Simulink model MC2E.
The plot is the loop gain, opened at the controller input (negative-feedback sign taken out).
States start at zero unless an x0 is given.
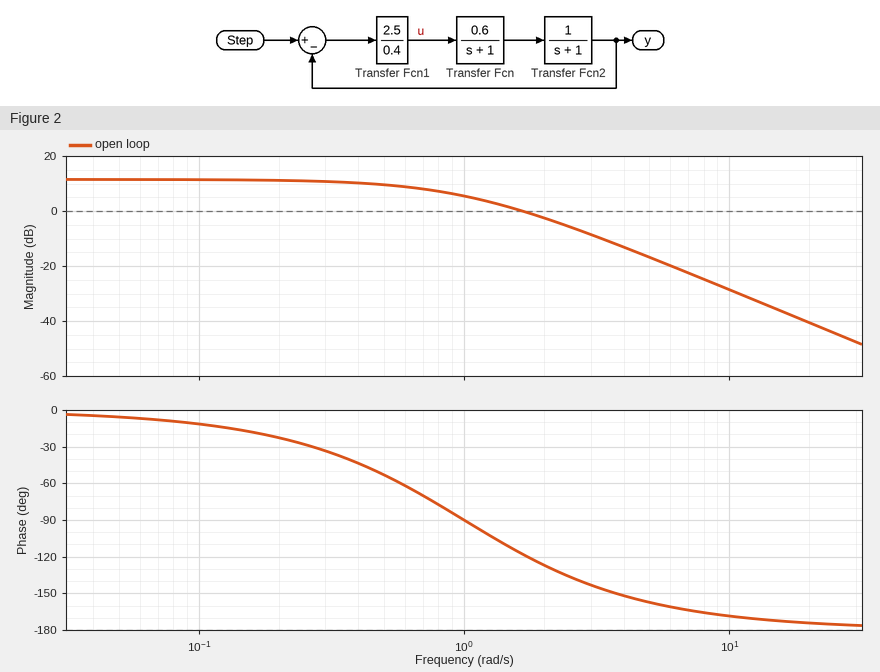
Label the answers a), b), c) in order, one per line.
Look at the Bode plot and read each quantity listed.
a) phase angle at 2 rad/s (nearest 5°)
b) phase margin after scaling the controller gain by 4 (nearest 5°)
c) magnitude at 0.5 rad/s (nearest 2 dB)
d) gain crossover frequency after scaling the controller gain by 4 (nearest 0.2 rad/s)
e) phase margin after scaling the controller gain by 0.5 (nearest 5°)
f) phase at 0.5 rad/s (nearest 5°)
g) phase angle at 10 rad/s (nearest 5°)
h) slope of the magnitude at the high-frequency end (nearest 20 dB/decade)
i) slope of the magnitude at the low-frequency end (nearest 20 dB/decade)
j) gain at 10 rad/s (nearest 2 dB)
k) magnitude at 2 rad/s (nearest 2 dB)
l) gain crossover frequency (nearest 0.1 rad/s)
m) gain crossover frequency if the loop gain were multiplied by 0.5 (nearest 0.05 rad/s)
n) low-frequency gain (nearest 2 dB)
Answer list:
a) -125°
b) 30°
c) 10 dB
d) 3.8 rad/s
e) 95°
f) -55°
g) -170°
h) -40 dB/decade
i) 0 dB/decade
j) -28 dB
k) -2 dB
l) 1.7 rad/s
m) 0.95 rad/s
n) 12 dB
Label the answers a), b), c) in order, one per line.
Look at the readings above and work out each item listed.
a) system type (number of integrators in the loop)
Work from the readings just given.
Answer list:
a) 0
